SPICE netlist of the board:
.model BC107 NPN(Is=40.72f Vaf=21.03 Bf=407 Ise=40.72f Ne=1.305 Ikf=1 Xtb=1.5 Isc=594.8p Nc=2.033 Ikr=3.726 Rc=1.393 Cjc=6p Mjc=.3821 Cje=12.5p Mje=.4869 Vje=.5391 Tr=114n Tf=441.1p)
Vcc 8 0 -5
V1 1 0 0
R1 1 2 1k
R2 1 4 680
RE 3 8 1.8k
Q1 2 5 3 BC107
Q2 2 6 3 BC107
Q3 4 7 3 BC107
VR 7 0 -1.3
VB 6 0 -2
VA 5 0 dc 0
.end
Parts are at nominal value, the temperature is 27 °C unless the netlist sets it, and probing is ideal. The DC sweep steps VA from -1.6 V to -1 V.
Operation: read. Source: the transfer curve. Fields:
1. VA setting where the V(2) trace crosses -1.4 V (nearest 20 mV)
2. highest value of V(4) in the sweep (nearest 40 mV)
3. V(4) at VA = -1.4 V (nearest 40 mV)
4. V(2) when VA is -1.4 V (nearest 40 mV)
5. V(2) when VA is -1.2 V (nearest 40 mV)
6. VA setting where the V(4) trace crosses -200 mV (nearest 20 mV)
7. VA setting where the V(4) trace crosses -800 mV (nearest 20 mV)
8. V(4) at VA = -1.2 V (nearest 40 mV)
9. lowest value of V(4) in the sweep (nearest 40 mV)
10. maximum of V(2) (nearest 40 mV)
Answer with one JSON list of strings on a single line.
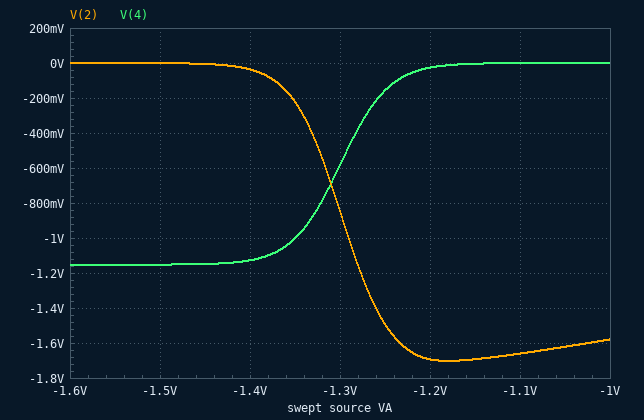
["-1.26 V", "0 V", "-1.12 V", "-40 mV", "-1.68 V", "-1.26 V", "-1.32 V", "-40 mV", "-1.16 V", "0 V"]
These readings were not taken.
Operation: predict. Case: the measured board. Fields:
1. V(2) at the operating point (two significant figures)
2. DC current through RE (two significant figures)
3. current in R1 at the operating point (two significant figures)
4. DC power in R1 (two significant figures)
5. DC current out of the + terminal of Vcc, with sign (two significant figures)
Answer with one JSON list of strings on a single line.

["-630 mV", "2.4 mA", "630 µA", "400 µW", "-2.4 mA"]
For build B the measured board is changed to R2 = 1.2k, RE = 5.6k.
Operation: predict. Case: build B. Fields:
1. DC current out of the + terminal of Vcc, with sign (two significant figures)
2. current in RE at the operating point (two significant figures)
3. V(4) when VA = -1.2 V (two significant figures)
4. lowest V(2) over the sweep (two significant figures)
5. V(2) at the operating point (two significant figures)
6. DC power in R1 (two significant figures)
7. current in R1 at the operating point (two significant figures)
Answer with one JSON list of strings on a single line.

["-780 µA", "780 µA", "-14 mV", "-600 mV", "-570 mV", "330 µW", "570 µA"]
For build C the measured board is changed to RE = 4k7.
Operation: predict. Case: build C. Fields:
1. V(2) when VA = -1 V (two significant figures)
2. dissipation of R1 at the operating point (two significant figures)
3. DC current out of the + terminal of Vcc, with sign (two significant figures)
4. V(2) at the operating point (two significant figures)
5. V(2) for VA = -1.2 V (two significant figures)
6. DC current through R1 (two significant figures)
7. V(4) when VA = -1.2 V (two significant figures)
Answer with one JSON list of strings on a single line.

["-720 mV", "340 µW", "-930 µA", "-590 mV", "-660 mV", "590 µA", "-9.7 mV"]
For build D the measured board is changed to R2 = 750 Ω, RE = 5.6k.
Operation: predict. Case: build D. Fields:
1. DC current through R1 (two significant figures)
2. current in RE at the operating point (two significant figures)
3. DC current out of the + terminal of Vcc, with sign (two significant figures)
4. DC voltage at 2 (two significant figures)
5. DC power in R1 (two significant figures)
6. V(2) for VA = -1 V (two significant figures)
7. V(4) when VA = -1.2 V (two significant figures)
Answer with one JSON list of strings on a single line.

["570 µA", "780 µA", "-780 µA", "-570 mV", "330 µW", "-600 mV", "-9.0 mV"]
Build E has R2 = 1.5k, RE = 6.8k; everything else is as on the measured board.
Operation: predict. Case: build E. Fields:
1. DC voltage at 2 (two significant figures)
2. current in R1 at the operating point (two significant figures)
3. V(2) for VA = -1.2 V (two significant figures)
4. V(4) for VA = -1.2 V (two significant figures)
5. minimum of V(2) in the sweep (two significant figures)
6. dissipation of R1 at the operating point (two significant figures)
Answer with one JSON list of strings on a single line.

["-550 mV", "550 µA", "-460 mV", "-15 mV", "-500 mV", "300 µW"]
